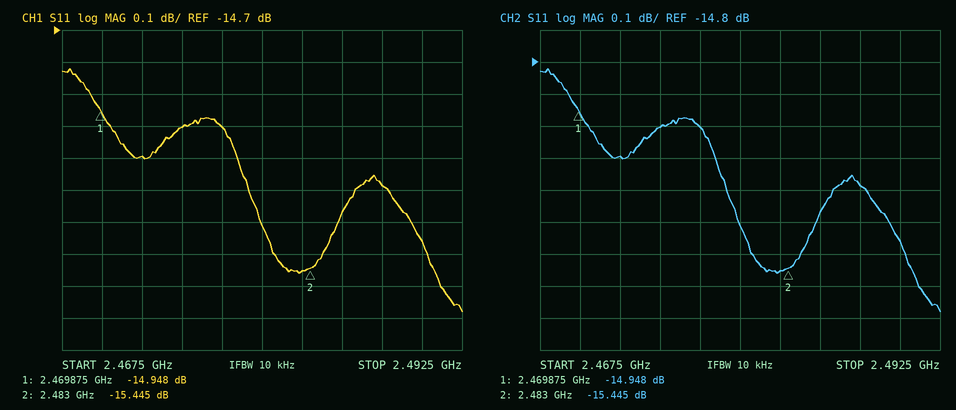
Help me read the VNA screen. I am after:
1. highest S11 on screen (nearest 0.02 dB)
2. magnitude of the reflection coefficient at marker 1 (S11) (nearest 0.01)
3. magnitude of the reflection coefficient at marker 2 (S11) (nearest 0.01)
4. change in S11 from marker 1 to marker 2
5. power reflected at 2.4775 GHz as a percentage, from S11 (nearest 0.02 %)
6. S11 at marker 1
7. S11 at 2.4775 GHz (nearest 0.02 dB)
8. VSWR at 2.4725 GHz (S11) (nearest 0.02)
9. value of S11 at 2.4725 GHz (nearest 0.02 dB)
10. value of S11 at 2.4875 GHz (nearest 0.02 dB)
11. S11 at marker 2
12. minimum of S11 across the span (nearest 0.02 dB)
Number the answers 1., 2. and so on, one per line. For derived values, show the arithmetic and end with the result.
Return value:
1. -14.82 dB
2. 10^(-14.948/20) ≈ 0.18
3. 10^(-15.445/20) ≈ 0.17
4. -15.445 − (-14.948) = -0.497 dB
5. 10^(-15/10) ≈ 3.16 %
6. -14.948 dB
7. -15.00 dB
8. |Γ| = 10^(-15.1/20) = 0.1758; VSWR = (1 + 0.1758)/(1 − 0.1758) ≈ 1.43, so 1.42 to the nearest 0.02
9. -15.10 dB
10. -15.18 dB
11. -15.445 dB
12. -15.58 dB
